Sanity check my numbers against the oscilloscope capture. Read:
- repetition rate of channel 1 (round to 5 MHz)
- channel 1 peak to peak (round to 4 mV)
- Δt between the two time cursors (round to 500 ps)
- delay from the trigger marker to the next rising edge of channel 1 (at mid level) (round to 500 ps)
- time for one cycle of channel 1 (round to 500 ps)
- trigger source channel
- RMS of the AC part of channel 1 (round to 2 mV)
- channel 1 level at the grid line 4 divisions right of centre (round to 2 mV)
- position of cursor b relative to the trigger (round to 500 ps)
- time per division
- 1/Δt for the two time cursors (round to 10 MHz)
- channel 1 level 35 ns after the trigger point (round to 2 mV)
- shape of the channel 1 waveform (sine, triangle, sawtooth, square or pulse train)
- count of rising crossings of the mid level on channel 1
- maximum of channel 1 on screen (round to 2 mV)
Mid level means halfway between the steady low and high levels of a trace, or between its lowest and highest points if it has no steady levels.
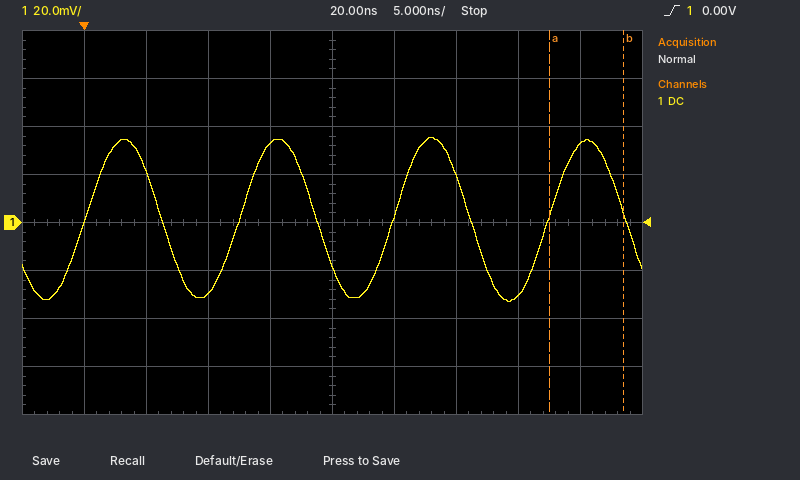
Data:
80 MHz
68 mV
6.0 ns
12.5 ns
12.5 ns
channel 1
24 mV
32 mV
+43.5 ns
5 ns
170 MHz
-30 mV
sine
4
36 mV
